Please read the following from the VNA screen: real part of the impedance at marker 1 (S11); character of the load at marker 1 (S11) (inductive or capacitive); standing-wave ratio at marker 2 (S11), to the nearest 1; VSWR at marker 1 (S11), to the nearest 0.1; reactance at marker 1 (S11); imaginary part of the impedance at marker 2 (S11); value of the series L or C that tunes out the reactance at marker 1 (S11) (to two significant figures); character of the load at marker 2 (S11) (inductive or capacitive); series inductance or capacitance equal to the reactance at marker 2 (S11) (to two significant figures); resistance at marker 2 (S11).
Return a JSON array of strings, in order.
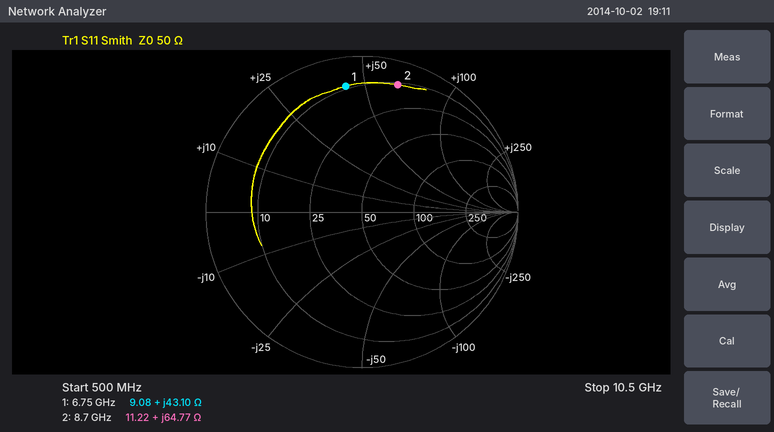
["9.08 Ω", "inductive", "12", "9.7", "+43.10 Ω", "+64.77 Ω", "550 fF", "inductive", "1.2 nH", "11.22 Ω"]
